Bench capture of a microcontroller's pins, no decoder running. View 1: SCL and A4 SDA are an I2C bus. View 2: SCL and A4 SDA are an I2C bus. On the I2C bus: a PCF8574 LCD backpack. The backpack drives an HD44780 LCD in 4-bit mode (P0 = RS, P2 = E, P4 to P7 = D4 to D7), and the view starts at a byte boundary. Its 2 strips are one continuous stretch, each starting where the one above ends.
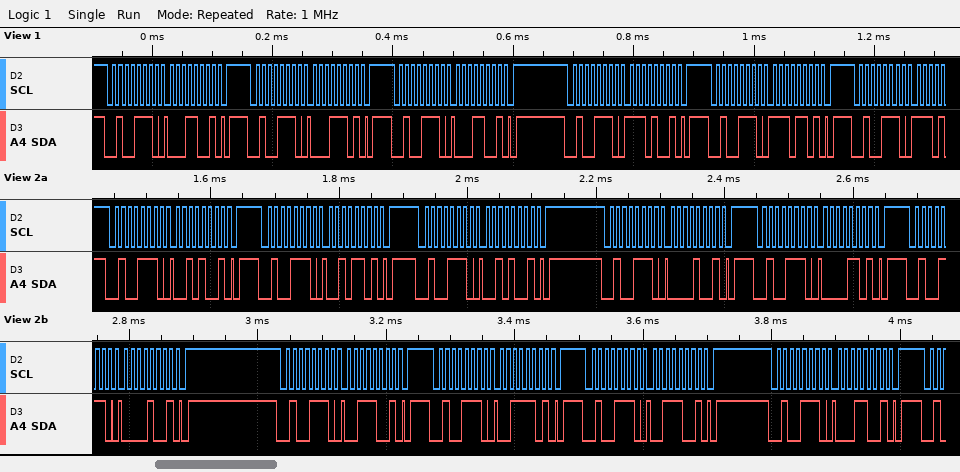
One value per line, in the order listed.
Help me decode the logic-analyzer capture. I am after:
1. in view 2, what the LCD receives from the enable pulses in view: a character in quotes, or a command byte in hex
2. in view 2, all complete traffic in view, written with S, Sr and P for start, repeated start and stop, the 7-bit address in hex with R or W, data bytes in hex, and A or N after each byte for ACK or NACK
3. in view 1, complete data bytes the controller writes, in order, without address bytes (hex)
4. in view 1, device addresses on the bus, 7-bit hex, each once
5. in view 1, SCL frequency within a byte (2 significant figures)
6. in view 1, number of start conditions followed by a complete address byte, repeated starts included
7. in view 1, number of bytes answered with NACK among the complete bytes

' '
S 27W A 29 A P S 27W A 2D A P S 27W A 29 A P S 27W A 09 A P S 27W A 0D A P S 27W A 09 A P S 27W A 39 A P S 27W A 3D A P S 27W A 39 A P S 27W A 19 A P
19 1D 19 E9 ED
0x27
100 kHz
6
0
